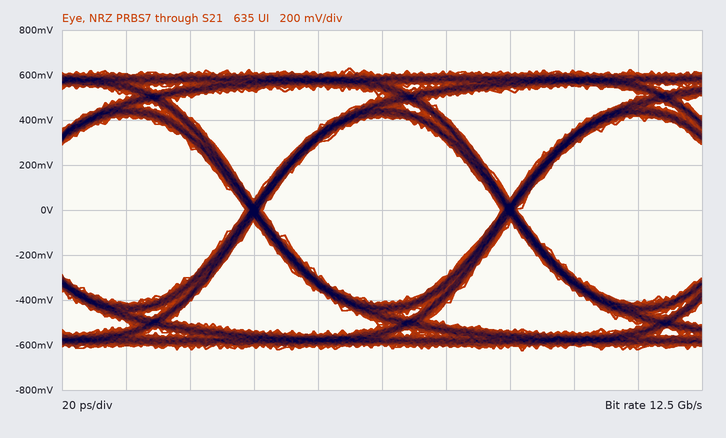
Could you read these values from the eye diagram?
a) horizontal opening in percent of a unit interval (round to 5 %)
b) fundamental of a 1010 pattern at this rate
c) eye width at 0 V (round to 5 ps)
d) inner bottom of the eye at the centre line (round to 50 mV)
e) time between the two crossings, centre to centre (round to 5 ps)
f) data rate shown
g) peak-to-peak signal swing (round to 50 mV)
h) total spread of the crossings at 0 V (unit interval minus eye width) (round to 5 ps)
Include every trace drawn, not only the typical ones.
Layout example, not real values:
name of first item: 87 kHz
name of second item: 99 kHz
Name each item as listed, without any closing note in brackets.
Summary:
horizontal opening in percent of a unit interval: 95 %
fundamental of a 1010 pattern at this rate: 6.25 GHz
eye width at 0 V: 75 ps
inner bottom of the eye at the centre line: -400 mV
time between the two crossings, centre to centre: 80 ps
data rate shown: 12.5 Gb/s
peak-to-peak signal swing: 1.25 V
total spread of the crossings at 0 V (unit interval minus eye width): 5 ps
